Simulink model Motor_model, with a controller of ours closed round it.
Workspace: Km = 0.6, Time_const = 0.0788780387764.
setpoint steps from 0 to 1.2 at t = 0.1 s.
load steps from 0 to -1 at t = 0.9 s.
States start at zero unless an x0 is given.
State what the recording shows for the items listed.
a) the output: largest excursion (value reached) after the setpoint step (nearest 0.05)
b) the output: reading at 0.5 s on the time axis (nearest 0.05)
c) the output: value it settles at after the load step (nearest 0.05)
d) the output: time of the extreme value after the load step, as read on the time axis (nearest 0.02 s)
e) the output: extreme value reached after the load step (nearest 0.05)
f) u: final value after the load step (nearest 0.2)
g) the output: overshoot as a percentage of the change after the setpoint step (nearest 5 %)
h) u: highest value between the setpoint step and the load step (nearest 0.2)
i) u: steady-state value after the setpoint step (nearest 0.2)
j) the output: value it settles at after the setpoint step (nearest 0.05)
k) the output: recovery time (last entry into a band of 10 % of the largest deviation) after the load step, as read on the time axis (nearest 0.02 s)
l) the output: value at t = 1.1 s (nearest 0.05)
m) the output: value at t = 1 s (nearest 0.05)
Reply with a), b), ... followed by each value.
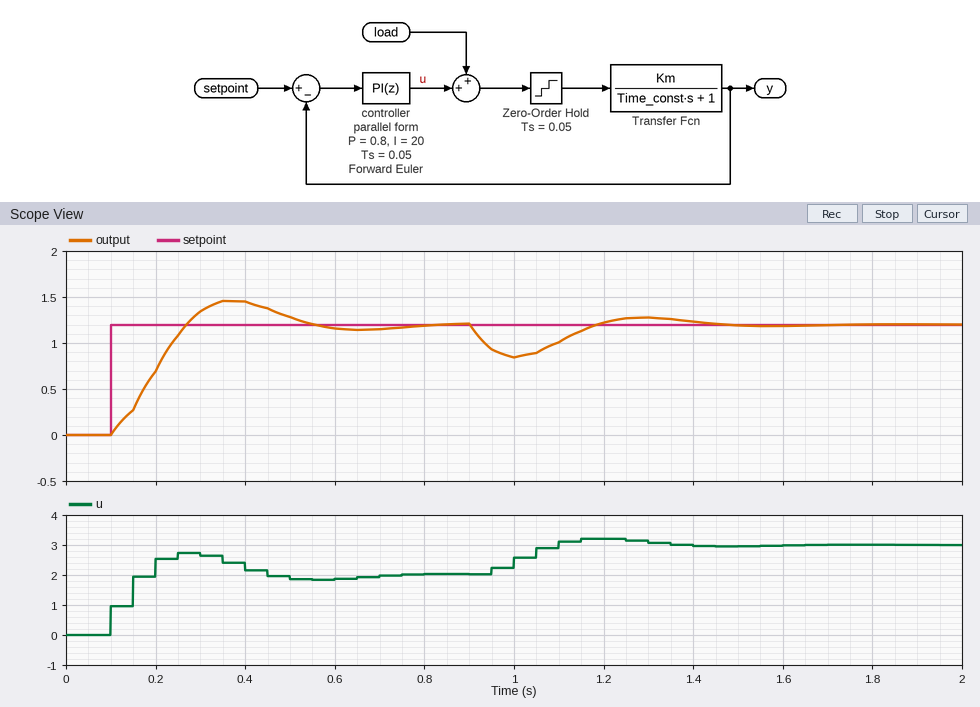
a) 1.45
b) 1.30
c) 1.20
d) 1.00 s
e) 0.85
f) 3.0
g) 20 %
h) 2.8
i) 2.0
j) 1.20
k) 1.40 s
l) 1.00
m) 0.85
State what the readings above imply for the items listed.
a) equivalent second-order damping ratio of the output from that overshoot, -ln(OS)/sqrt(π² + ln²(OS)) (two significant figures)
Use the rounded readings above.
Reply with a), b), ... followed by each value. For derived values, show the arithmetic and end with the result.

a) ln(0.2) = -1.609; 1.609 / sqrt(9.870 + 2.590) = 0.46
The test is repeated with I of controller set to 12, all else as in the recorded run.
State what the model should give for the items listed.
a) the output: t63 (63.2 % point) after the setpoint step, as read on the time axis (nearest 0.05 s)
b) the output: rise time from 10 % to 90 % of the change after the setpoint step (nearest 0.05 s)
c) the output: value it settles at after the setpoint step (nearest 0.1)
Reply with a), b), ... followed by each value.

a) 0.25 s
b) 0.20 s
c) 1.2
